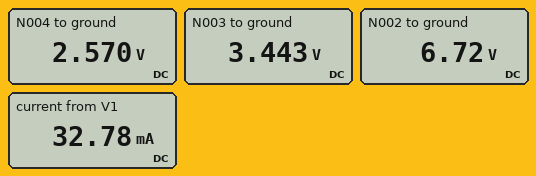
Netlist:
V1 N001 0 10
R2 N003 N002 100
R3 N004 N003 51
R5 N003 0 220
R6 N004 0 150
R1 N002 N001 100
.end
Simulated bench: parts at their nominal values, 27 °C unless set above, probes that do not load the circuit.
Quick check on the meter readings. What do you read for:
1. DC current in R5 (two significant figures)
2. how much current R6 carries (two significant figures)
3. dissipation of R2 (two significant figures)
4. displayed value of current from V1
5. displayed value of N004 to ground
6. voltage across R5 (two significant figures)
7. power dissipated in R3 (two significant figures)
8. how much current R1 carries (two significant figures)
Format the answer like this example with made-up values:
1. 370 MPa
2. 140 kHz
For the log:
1. 16 mA
2. 17 mA
3. 110 mW
4. 32.78 mA
5. 2.570 V
6. 3.4 V
7. 15 mW
8. 33 mA
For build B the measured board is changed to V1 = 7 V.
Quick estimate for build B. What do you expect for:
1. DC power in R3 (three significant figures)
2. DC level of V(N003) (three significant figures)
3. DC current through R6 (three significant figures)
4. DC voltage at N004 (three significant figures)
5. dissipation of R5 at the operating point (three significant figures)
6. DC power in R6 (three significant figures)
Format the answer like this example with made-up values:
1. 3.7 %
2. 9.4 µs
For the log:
1. 7.33 mW
2. 2.41 V
3. 12.0 mA
4. 1.80 V
5. 26.4 mW
6. 21.6 mW
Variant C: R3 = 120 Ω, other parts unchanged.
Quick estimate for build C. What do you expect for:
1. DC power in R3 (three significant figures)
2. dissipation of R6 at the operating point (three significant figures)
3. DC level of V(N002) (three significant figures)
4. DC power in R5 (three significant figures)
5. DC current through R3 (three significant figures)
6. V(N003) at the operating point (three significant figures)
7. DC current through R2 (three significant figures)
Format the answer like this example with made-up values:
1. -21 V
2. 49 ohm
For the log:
1. 23.4 mW
2. 29.3 mW
3. 6.89 V
4. 64.7 mW
5. 14.0 mA
6. 3.77 V
7. 31.1 mA
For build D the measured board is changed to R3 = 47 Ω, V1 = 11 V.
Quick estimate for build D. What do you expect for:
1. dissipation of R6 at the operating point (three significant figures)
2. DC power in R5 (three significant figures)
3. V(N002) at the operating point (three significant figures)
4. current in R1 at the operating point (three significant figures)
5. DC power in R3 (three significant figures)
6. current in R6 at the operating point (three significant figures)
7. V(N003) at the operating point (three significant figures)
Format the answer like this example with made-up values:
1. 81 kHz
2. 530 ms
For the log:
1. 54.7 mW
2. 64.3 mW
3. 7.38 V
4. 36.2 mA
5. 17.1 mW
6. 19.1 mA
7. 3.76 V
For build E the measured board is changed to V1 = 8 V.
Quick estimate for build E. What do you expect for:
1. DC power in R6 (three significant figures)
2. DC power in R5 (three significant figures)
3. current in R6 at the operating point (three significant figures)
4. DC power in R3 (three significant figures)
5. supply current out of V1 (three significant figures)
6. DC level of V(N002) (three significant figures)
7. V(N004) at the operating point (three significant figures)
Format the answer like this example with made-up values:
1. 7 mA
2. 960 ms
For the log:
1. 28.2 mW
2. 34.5 mW
3. 13.7 mA
4. 9.58 mW
5. 26.2 mA
6. 5.38 V
7. 2.06 V
